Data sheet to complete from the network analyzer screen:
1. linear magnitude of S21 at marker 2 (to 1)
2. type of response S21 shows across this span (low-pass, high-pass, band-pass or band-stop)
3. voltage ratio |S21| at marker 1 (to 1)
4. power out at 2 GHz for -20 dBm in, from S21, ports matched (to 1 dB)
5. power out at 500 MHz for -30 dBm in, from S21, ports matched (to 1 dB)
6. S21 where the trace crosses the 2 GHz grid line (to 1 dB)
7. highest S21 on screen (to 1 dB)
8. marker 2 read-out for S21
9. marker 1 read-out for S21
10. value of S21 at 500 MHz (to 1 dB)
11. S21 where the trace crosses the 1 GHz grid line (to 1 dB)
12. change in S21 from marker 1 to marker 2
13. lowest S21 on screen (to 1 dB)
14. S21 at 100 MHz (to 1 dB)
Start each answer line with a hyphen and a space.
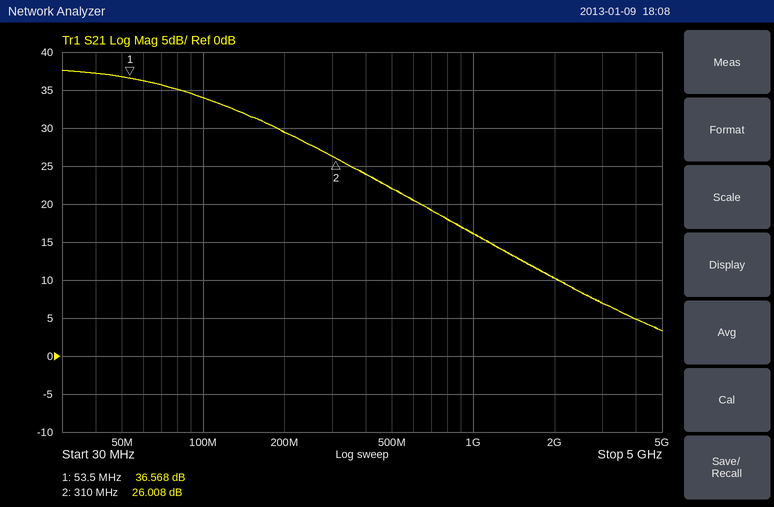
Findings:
- 20
- low-pass
- 67
- -10 dBm
- -8 dBm
- 10 dB
- 38 dB
- 26.008 dB
- 36.568 dB
- 22 dB
- 16 dB
- -10.560 dB
- 3 dB
- 34 dB
